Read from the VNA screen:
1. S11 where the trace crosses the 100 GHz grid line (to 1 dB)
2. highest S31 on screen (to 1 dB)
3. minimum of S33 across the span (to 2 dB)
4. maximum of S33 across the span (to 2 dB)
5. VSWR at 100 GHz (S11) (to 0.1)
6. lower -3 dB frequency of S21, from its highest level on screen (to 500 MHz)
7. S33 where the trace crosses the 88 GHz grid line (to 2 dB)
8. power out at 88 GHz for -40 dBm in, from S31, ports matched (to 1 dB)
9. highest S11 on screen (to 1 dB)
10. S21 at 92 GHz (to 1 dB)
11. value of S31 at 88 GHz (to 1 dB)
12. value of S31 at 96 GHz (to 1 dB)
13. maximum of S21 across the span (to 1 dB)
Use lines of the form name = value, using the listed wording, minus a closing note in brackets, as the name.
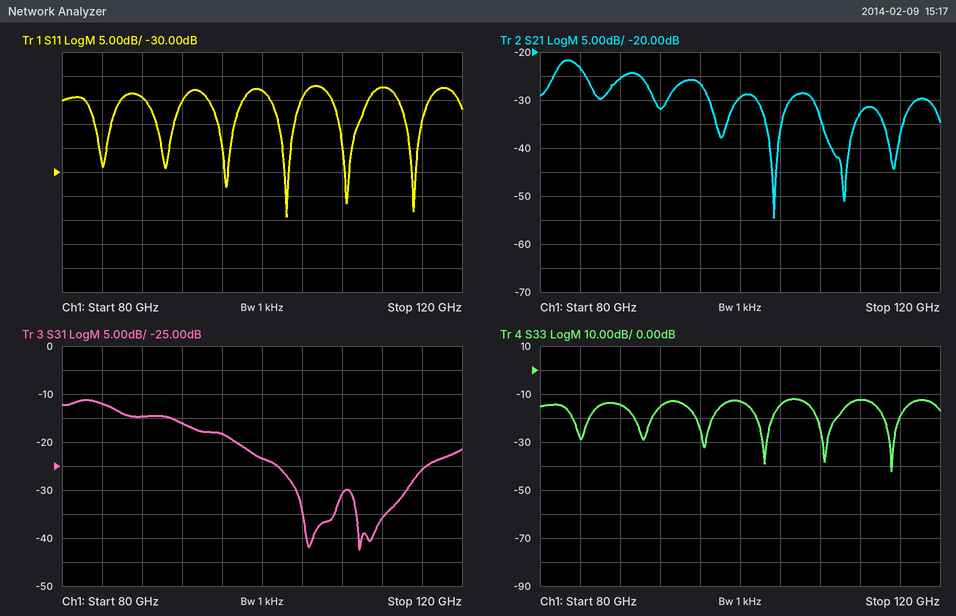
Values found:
S11 where the trace crosses the 100 GHz grid line = -13 dB
highest S31 on screen = -11 dB
minimum of S33 across the span = -42 dB
maximum of S33 across the span = -12 dB
VSWR at 100 GHz (S11) = 1.6
lower -3 dB frequency of S21, from its highest level on screen = 81.5 GHz
S33 where the trace crosses the 88 GHz grid line = -14 dB
power out at 88 GHz for -40 dBm in, from S31, ports matched = -55 dBm
highest S11 on screen = -12 dB
S21 at 92 GHz = -32 dB
value of S31 at 88 GHz = -15 dB
value of S31 at 96 GHz = -18 dB
maximum of S21 across the span = -22 dB
